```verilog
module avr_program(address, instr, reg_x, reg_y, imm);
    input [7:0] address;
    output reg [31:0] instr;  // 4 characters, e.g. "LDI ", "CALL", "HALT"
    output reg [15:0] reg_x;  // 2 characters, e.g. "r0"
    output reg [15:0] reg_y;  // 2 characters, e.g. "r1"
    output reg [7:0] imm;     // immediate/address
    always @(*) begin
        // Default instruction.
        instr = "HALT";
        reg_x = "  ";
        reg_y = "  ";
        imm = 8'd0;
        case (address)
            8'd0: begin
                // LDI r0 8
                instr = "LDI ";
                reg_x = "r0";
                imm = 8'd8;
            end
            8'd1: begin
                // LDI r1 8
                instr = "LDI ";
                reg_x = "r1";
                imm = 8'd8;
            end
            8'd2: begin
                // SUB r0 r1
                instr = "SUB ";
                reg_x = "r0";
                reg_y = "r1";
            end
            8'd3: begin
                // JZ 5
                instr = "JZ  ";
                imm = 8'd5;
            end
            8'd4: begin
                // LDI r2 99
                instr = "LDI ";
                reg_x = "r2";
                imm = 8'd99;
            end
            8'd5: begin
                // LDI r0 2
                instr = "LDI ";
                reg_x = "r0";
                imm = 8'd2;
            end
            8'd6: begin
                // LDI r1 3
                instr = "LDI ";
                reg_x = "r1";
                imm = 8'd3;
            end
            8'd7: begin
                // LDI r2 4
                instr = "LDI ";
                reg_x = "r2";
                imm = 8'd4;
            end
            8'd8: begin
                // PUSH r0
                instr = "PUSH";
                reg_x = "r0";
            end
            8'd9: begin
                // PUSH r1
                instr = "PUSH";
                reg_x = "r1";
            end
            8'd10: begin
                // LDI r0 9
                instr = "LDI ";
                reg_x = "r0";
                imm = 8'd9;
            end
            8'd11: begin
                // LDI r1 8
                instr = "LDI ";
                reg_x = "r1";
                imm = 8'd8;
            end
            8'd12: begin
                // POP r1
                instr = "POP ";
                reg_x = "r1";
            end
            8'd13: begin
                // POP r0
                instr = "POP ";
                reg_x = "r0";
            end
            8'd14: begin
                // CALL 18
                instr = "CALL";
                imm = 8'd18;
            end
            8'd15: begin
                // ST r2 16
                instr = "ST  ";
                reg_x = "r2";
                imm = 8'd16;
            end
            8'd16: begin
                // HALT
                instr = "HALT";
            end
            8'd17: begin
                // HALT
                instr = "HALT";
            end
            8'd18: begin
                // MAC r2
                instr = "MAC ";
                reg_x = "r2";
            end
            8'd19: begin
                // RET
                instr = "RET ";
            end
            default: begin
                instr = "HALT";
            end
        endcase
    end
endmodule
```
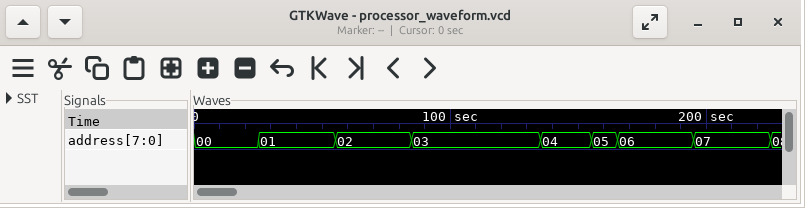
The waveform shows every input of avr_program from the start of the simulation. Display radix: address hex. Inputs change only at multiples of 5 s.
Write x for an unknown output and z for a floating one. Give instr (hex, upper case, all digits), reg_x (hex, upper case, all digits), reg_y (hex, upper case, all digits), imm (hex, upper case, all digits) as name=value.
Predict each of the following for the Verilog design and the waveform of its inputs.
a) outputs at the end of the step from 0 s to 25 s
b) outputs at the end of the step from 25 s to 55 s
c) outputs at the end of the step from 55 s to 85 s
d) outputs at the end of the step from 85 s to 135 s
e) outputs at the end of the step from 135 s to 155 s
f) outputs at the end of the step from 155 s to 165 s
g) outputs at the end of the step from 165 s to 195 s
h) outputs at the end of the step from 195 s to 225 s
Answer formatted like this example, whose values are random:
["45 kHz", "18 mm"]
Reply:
["instr=4C444920, reg_x=7230, reg_y=2020, imm=08", "instr=4C444920, reg_x=7231, reg_y=2020, imm=08", "instr=53554220, reg_x=7230, reg_y=7231, imm=00", "instr=4A5A2020, reg_x=2020, reg_y=2020, imm=05", "instr=4C444920, reg_x=7232, reg_y=2020, imm=63", "instr=4C444920, reg_x=7230, reg_y=2020, imm=02", "instr=4C444920, reg_x=7231, reg_y=2020, imm=03", "instr=4C444920, reg_x=7232, reg_y=2020, imm=04"]
